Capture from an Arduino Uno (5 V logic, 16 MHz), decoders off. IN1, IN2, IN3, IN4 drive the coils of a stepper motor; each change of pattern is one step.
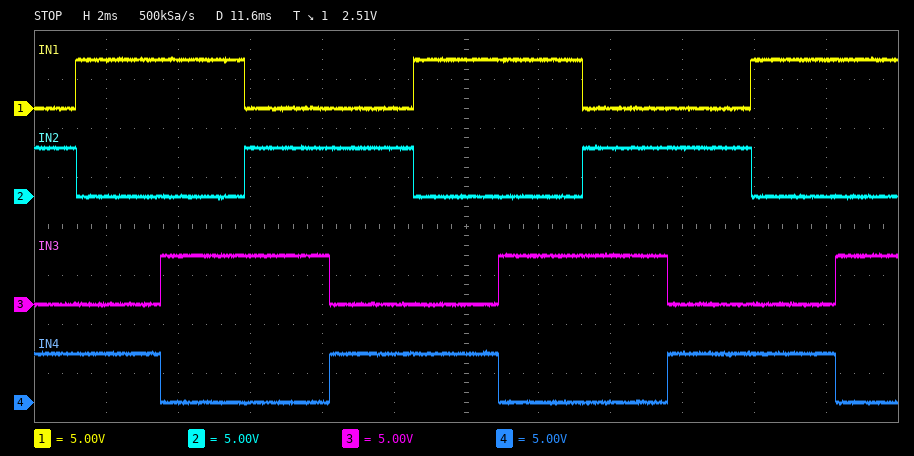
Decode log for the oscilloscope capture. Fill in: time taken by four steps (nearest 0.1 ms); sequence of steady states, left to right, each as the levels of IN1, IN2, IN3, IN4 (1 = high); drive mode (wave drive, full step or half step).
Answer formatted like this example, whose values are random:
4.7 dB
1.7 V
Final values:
9.4 ms
0101 1001 1010 0110 0101 1001 1010 0110 0101 1001 1010
full step
